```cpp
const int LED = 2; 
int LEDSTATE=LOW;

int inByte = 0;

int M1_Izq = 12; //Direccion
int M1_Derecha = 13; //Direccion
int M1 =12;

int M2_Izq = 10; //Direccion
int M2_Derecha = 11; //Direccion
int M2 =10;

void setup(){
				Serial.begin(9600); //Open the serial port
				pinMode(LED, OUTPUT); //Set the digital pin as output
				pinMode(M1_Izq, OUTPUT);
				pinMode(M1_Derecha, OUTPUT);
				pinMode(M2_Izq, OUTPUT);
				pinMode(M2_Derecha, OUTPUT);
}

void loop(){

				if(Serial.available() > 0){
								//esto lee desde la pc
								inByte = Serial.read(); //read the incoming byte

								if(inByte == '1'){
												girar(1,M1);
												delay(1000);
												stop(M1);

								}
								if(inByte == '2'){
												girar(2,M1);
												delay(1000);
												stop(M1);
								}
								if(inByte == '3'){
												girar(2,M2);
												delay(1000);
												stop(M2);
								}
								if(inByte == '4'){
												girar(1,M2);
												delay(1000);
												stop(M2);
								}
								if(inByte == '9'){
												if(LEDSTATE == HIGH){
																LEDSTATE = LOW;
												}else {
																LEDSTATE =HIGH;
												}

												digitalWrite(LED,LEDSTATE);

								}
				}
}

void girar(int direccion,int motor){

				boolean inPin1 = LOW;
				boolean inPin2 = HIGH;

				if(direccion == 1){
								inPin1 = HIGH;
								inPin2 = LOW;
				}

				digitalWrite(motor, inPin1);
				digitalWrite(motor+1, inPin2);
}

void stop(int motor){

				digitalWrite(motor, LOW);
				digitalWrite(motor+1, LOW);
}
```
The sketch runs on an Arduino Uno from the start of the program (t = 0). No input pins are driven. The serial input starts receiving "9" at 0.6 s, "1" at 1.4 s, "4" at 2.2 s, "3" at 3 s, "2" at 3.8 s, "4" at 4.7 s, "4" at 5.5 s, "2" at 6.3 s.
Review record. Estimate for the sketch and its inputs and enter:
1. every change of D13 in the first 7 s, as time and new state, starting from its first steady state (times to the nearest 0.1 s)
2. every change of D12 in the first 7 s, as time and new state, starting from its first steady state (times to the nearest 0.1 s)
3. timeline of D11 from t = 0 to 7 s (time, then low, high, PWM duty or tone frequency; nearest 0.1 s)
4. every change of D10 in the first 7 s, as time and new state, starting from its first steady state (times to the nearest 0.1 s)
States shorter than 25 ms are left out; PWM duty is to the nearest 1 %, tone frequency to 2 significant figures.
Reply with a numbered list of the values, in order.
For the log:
1. 0 s low; 4.4 s high; 5.4 s low
2. 0 s low; 1.4 s high; 2.4 s low
3. 0 s low; 3.4 s high; 4.4 s low
4. 0 s low; 2.4 s high; 3.4 s low; 5.4 s high
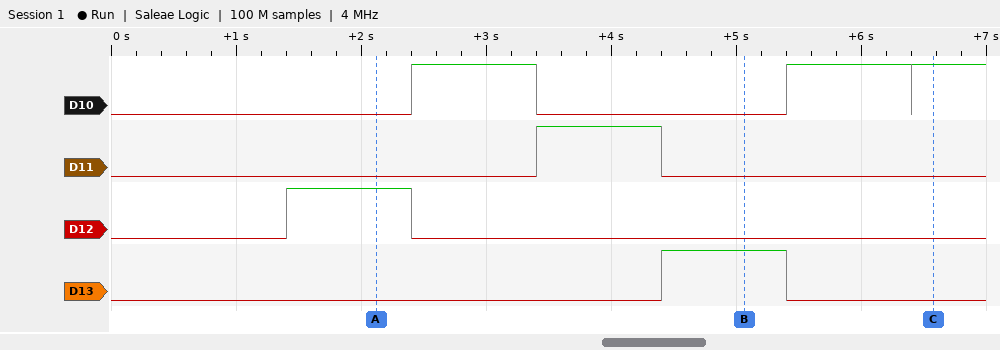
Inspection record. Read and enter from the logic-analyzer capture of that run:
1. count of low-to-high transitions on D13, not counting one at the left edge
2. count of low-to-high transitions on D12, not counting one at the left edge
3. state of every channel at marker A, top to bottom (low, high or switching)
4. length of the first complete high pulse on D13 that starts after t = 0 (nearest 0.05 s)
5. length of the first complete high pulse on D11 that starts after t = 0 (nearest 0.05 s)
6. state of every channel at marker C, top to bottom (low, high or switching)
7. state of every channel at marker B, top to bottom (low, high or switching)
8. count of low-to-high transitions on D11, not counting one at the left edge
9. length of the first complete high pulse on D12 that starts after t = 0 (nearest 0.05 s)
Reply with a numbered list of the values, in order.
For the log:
1. 1
2. 1
3. D10 low, D11 low, D12 high, D13 low
4. 1.00 s
5. 1.00 s
6. D10 high, D11 low, D12 low, D13 low
7. D10 low, D11 low, D12 low, D13 high
8. 1
9. 1.00 s
